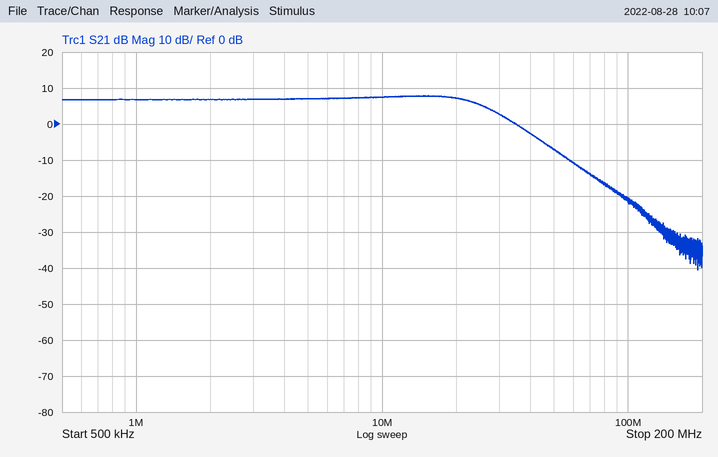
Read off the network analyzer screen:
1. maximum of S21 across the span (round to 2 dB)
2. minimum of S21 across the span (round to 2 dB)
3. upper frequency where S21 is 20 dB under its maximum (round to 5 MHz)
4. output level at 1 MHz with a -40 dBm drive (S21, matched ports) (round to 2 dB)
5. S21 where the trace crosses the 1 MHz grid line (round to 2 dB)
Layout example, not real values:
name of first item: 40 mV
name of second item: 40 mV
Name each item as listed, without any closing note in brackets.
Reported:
maximum of S21 across the span: 8 dB
minimum of S21 across the span: -40 dB
upper frequency where S21 is 20 dB under its maximum: 65 MHz
output level at 1 MHz with a -40 dBm drive (S21, matched ports): -34 dBm
S21 where the trace crosses the 1 MHz grid line: 6 dB
